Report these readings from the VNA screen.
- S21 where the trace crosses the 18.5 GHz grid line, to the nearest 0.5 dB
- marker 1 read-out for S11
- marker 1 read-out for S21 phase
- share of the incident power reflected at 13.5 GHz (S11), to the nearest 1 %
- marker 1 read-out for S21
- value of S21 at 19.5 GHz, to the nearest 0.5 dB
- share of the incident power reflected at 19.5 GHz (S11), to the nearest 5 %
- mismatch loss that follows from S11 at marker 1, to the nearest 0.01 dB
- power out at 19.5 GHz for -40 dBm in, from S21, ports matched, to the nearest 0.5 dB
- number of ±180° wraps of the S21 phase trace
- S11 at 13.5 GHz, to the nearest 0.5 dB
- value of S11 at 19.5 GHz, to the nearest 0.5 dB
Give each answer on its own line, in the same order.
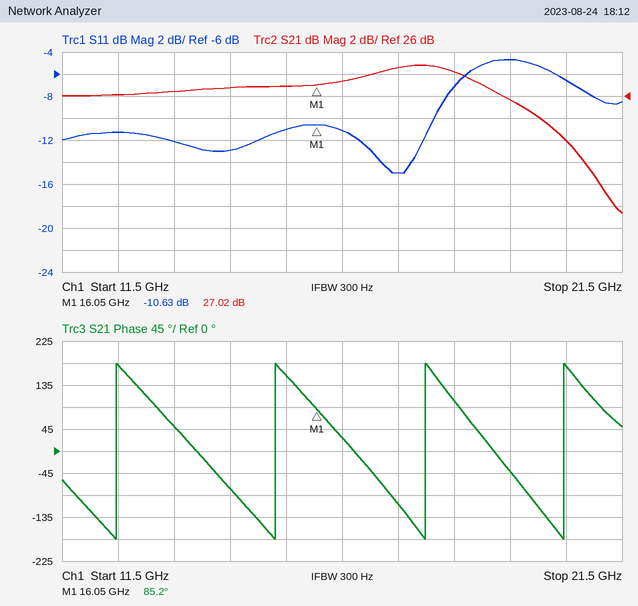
28.0 dB
-10.63 dB
85.2°
6 %
27.02 dB
25.5 dB
35 %
0.39 dB
-14.5 dBm
4
-12.0 dB
-4.5 dB
